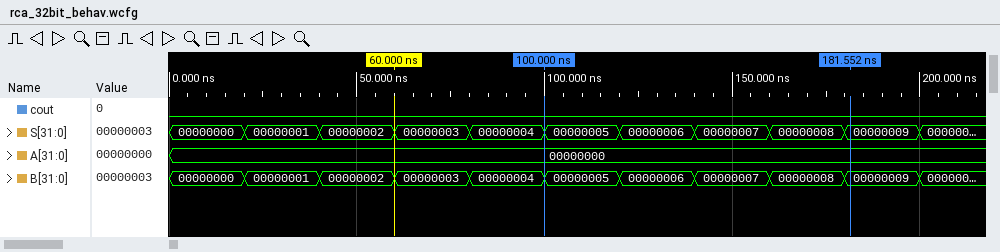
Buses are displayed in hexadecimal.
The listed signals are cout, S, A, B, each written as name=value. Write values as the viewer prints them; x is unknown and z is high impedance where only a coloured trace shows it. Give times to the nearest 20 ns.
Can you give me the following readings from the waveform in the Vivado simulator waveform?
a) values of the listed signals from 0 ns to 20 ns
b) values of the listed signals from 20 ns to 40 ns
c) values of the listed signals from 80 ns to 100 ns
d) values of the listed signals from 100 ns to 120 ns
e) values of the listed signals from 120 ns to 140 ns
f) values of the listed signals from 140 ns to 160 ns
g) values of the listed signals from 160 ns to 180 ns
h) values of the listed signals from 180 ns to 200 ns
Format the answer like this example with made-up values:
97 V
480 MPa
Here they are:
cout=0, S=00000000, A=00000000, B=00000000
cout=0, S=00000001, A=00000000, B=00000001
cout=0, S=00000004, A=00000000, B=00000004
cout=0, S=00000005, A=00000000, B=00000005
cout=0, S=00000006, A=00000000, B=00000006
cout=0, S=00000007, A=00000000, B=00000007
cout=0, S=00000008, A=00000000, B=00000008
cout=0, S=00000009, A=00000000, B=00000009
